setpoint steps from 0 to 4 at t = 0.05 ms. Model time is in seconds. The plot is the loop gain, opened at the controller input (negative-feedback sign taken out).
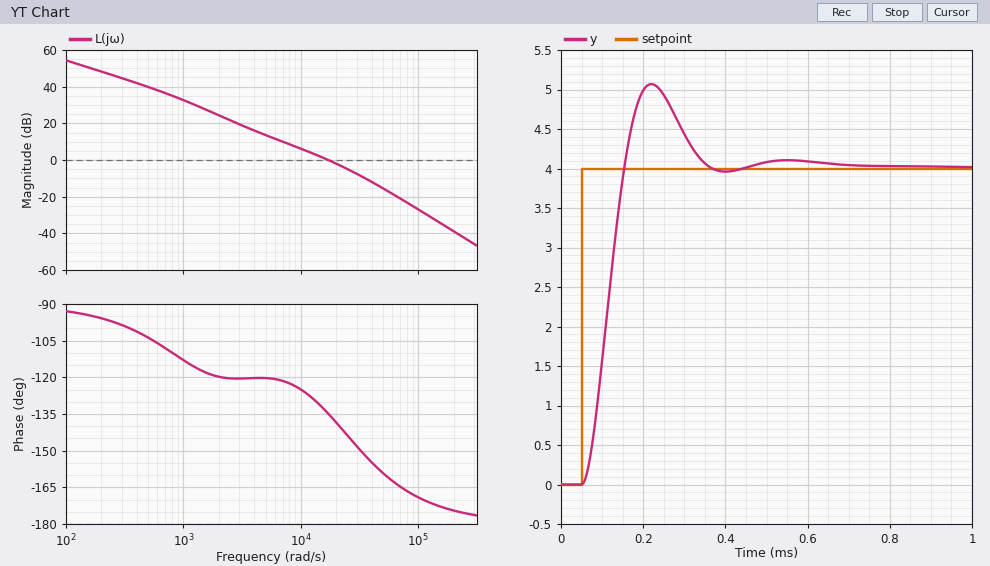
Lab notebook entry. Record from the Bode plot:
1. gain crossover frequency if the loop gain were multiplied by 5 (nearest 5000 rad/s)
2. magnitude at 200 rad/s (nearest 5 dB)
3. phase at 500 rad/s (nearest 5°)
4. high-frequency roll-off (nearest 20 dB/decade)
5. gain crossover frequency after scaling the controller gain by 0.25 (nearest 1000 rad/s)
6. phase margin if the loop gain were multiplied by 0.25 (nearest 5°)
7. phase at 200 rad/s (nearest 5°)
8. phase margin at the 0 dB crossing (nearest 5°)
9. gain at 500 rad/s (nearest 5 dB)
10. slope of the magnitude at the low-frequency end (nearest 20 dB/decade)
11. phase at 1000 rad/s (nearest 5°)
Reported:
45000 rad/s
50 dB
-105°
-40 dB/decade
6000 rad/s
60°
-95°
45°
40 dB
-20 dB/decade
-115°
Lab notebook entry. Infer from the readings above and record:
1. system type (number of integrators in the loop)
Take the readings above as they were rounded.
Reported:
1
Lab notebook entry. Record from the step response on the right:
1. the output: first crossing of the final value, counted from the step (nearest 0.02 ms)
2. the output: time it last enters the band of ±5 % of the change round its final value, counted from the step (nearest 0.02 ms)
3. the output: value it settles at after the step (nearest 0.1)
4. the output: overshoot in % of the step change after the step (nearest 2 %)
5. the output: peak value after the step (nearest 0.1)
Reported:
0.10 ms
0.28 ms
4.0
26 %
5.1
